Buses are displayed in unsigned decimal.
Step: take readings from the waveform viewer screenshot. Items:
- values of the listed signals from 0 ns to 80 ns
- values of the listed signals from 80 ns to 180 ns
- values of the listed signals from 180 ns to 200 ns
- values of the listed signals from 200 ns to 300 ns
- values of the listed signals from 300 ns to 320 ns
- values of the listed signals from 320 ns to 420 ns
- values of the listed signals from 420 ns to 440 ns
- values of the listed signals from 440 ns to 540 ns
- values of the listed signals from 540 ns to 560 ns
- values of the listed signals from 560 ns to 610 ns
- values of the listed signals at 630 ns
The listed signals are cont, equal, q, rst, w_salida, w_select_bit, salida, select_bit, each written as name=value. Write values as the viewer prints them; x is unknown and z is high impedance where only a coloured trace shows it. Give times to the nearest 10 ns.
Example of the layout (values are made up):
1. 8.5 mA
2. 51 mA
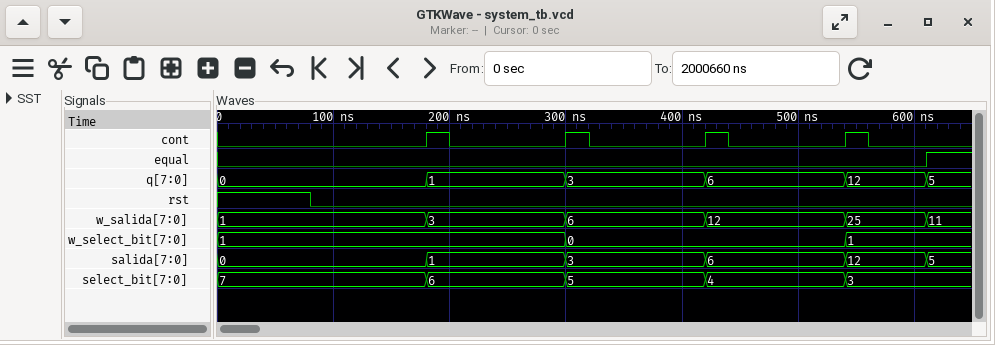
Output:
1. cont=0, equal=0, q=0, rst=1, w_salida=1, w_select_bit=1, salida=0, select_bit=7
2. cont=0, equal=0, q=0, rst=0, w_salida=1, w_select_bit=1, salida=0, select_bit=7
3. cont=1, equal=0, q=1, rst=0, w_salida=3, w_select_bit=1, salida=1, select_bit=6
4. cont=0, equal=0, q=1, rst=0, w_salida=3, w_select_bit=1, salida=1, select_bit=6
5. cont=1, equal=0, q=3, rst=0, w_salida=6, w_select_bit=0, salida=3, select_bit=5
6. cont=0, equal=0, q=3, rst=0, w_salida=6, w_select_bit=0, salida=3, select_bit=5
7. cont=1, equal=0, q=6, rst=0, w_salida=12, w_select_bit=0, salida=6, select_bit=4
8. cont=0, equal=0, q=6, rst=0, w_salida=12, w_select_bit=0, salida=6, select_bit=4
9. cont=1, equal=0, q=12, rst=0, w_salida=25, w_select_bit=1, salida=12, select_bit=3
10. cont=0, equal=0, q=12, rst=0, w_salida=25, w_select_bit=1, salida=12, select_bit=3
11. cont=0, equal=1, q=5, rst=0, w_salida=11, w_select_bit=1, salida=5, select_bit=3
